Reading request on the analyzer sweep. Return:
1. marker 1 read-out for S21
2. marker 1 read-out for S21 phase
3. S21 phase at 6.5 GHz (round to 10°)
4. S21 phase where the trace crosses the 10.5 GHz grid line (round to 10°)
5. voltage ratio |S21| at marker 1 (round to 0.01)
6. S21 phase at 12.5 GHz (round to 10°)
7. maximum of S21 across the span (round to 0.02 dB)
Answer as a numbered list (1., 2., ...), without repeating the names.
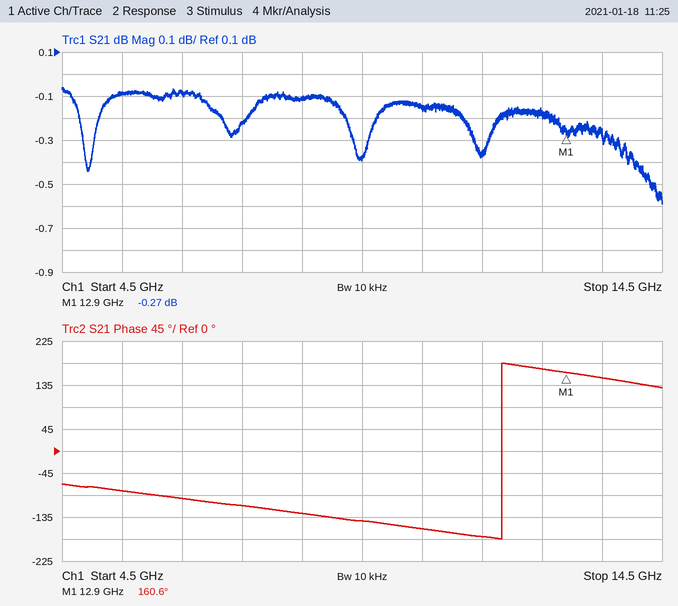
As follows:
1. -0.27 dB
2. 160.6°
3. -100°
4. -160°
5. 0.97
6. 170°
7. -0.06 dB
